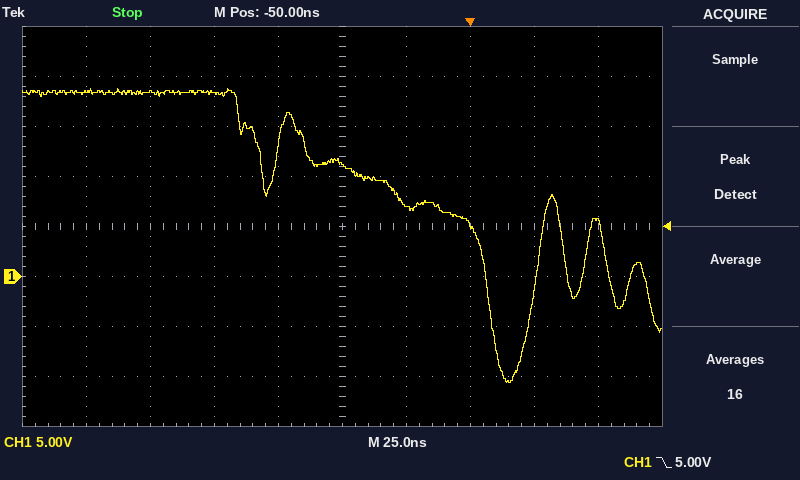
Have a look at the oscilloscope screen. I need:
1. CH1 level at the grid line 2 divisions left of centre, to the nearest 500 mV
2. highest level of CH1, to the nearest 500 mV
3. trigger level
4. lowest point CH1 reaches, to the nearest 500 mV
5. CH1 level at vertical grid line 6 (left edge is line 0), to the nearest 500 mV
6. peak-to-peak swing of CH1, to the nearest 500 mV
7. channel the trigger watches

18.5 V
19.0 V
5.00 V
-10.5 V
7.0 V
29.5 V
CH1
